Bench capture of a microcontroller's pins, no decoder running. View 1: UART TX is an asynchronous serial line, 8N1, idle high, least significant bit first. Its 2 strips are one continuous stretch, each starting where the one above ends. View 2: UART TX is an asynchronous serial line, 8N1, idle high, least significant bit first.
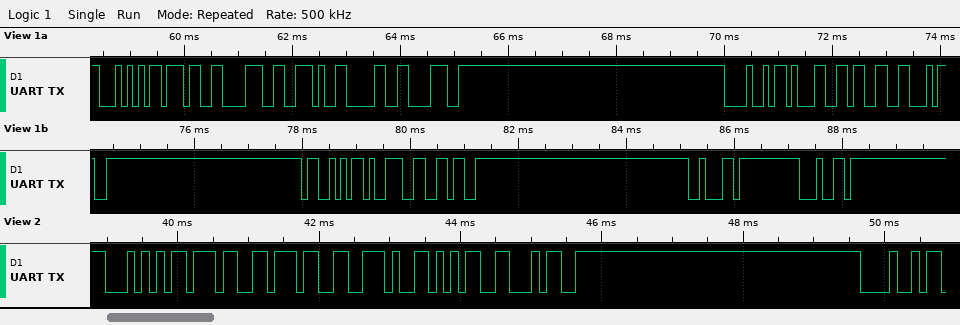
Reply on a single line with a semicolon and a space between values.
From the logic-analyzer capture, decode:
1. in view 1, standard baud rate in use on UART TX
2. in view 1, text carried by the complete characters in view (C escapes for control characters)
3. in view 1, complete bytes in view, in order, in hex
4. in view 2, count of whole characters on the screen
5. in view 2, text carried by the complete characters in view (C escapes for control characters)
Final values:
9600 baud; "T78.08H134S96bd"; 54 37 38 2E 30 38 48 31 33 34 53 39 36 62 64; 7; "T77.54H"
